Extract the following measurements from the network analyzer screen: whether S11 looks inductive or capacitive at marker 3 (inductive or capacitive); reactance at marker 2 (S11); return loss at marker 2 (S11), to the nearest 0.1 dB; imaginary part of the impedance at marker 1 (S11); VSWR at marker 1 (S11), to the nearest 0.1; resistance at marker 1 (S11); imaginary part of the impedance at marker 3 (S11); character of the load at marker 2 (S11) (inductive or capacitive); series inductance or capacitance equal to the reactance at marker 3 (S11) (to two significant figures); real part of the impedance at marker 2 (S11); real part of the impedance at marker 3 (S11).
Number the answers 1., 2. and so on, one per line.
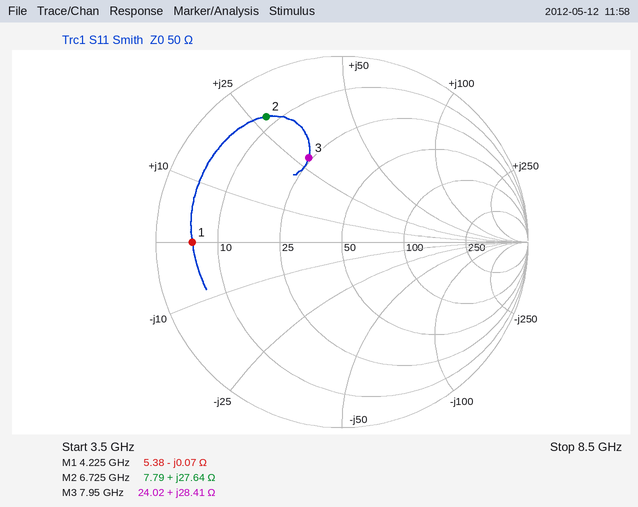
1. inductive
2. +27.64 Ω
3. 2.1 dB
4. -0.07 Ω
5. 9.3
6. 5.38 Ω
7. +28.41 Ω
8. inductive
9. 570 pH
10. 7.79 Ω
11. 24.02 Ω
